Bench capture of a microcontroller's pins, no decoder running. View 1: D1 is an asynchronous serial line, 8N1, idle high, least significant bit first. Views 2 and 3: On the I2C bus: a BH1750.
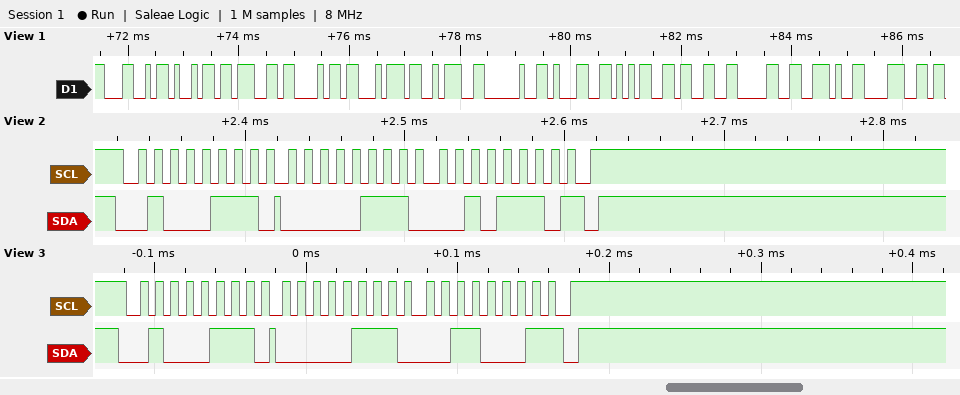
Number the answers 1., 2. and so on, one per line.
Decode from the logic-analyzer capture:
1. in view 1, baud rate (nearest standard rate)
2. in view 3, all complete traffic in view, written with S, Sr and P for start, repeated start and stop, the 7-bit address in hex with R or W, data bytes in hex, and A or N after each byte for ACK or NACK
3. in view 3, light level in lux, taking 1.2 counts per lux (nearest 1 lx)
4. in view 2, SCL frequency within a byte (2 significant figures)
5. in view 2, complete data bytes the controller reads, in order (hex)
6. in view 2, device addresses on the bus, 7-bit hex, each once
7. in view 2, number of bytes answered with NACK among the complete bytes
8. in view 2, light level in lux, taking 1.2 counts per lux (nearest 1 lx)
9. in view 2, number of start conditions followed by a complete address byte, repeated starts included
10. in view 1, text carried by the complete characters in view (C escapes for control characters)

1. 9600 baud
2. S 23R A 07 A 31 N P
3. 1534 lx
4. 100 kHz
5. 07 2E
6. 0x23
7. 1
8. 1532 lx
9. 1
10. "Light: 1530.8"
